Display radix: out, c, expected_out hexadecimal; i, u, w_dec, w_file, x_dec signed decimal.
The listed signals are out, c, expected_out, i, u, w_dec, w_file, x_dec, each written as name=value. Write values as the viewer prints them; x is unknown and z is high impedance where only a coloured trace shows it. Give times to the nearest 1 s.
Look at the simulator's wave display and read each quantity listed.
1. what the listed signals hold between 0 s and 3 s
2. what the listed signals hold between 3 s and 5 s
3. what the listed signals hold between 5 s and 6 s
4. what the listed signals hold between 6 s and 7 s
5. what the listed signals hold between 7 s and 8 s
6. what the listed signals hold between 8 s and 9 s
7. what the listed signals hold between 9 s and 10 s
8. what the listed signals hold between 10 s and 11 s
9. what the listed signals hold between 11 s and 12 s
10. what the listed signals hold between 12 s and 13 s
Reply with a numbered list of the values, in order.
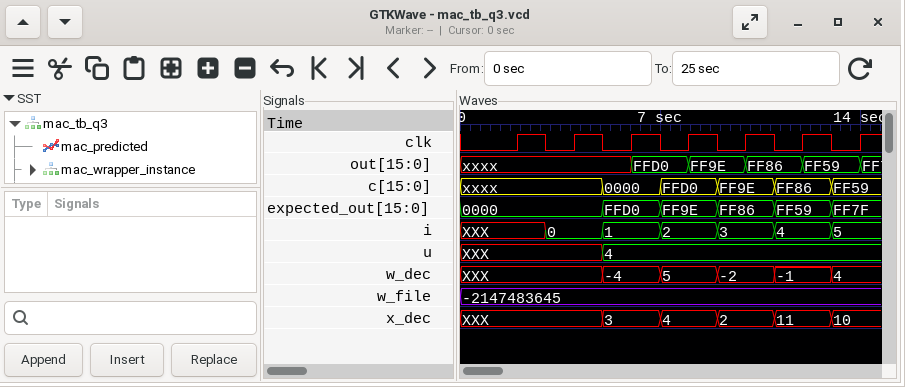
1. out=xxxx, c=xxxx, expected_out=0000, i=XXX, u=XXX, w_dec=XXX, w_file=-2147483645, x_dec=XXX
2. out=xxxx, c=xxxx, expected_out=0000, i=0, u=XXX, w_dec=XXX, w_file=-2147483645, x_dec=XXX
3. out=xxxx, c=0000, expected_out=FFD0, i=1, u=4, w_dec=-4, w_file=-2147483645, x_dec=3
4. out=FFD0, c=0000, expected_out=FFD0, i=1, u=4, w_dec=-4, w_file=-2147483645, x_dec=3
5. out=FFD0, c=FFD0, expected_out=FF9E, i=2, u=4, w_dec=5, w_file=-2147483645, x_dec=4
6. out=FF9E, c=FFD0, expected_out=FF9E, i=2, u=4, w_dec=5, w_file=-2147483645, x_dec=4
7. out=FF9E, c=FF9E, expected_out=FF86, i=3, u=4, w_dec=-2, w_file=-2147483645, x_dec=2
8. out=FF86, c=FF9E, expected_out=FF86, i=3, u=4, w_dec=-2, w_file=-2147483645, x_dec=2
9. out=FF86, c=FF86, expected_out=FF59, i=4, u=4, w_dec=-1, w_file=-2147483645, x_dec=11
10. out=FF59, c=FF86, expected_out=FF59, i=4, u=4, w_dec=-1, w_file=-2147483645, x_dec=11
